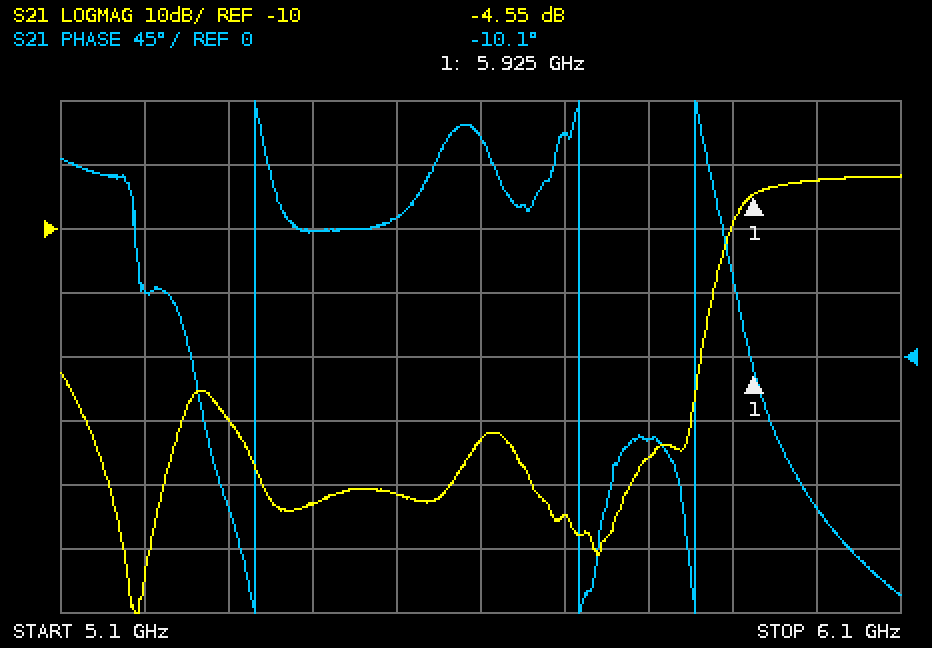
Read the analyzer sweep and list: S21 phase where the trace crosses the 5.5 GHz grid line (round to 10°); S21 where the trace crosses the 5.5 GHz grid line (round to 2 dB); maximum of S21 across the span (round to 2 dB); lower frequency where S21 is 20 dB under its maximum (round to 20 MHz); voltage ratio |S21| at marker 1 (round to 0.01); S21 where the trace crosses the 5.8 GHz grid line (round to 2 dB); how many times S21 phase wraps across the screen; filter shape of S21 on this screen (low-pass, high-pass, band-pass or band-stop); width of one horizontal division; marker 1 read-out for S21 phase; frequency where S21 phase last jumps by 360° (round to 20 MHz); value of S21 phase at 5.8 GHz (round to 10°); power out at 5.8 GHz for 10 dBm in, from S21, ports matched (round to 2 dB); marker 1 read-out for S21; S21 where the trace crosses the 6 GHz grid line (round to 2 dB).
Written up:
100°
-52 dB
-2 dB
5.88 GHz
0.59
-46 dB
3
high-pass
100 MHz
-10.1°
5.86 GHz
-60°
-36 dBm
-4.55 dB
-2 dB
